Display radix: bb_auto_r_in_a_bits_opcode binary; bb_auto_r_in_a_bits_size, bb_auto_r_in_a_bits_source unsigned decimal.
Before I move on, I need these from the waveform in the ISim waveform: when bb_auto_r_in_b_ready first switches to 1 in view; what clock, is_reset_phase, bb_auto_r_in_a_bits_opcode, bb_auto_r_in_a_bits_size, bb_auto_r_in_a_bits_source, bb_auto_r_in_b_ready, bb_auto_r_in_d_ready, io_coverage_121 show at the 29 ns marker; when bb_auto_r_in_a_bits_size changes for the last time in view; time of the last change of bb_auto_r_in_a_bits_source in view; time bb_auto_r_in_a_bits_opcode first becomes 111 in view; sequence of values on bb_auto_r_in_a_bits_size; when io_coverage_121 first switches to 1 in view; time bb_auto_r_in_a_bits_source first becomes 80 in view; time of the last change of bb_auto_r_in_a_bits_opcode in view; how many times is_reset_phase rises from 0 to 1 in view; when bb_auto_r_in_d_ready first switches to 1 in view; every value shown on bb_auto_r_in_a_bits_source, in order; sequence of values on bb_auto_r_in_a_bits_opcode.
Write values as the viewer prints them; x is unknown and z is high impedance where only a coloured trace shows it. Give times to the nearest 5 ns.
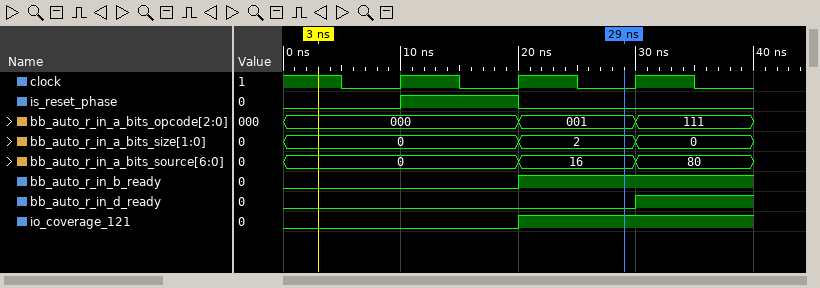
20 ns
clock=0, is_reset_phase=0, bb_auto_r_in_a_bits_opcode=001, bb_auto_r_in_a_bits_size=2, bb_auto_r_in_a_bits_source=16, bb_auto_r_in_b_ready=1, bb_auto_r_in_d_ready=0, io_coverage_121=1
30 ns
30 ns
30 ns
0, 2, 0
20 ns
30 ns
30 ns
1
30 ns
0, 16, 80
000, 001, 111
